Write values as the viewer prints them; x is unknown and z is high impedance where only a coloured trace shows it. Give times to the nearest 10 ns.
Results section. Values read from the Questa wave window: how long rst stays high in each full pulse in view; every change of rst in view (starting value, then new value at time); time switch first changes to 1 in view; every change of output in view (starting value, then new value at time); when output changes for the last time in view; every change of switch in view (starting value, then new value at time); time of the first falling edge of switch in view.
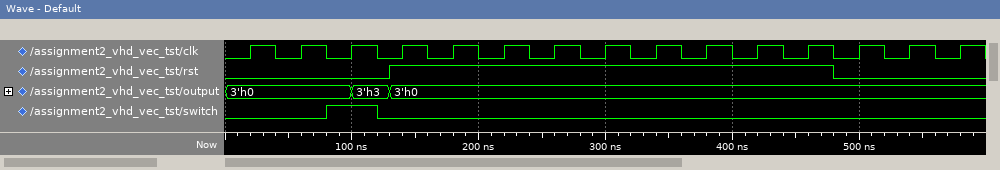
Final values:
350 ns
0, 1 at 130 ns, 0 at 480 ns
80 ns
3'h0, 3'h3 at 100 ns, 3'h0 at 130 ns
130 ns
0, 1 at 80 ns, 0 at 120 ns
120 ns
